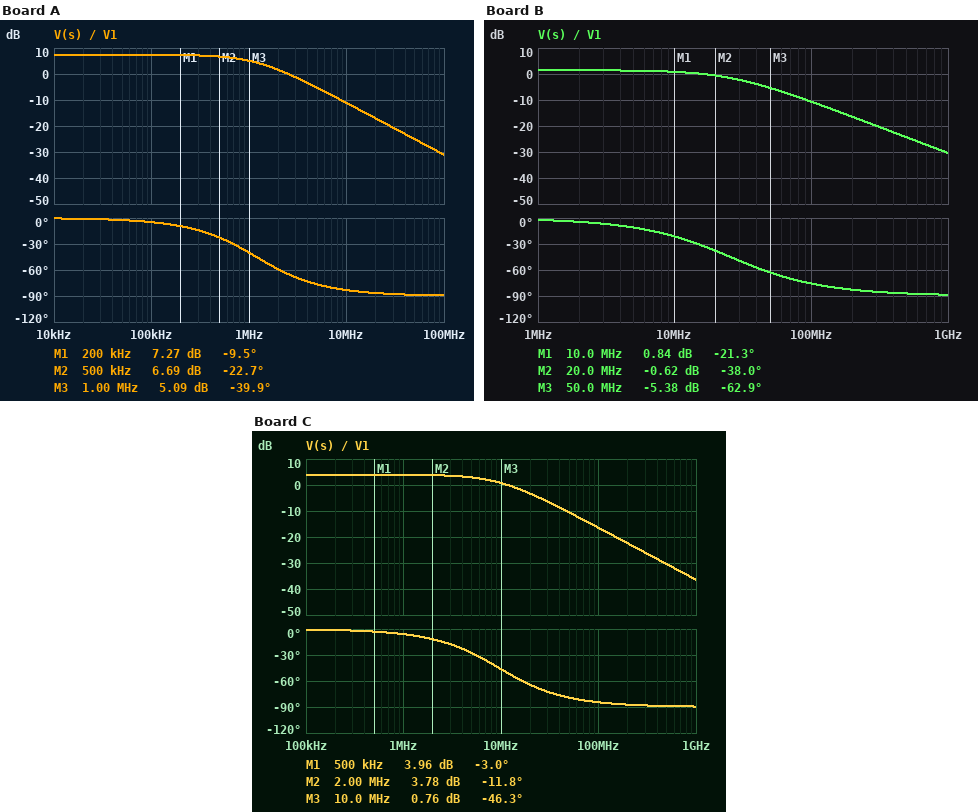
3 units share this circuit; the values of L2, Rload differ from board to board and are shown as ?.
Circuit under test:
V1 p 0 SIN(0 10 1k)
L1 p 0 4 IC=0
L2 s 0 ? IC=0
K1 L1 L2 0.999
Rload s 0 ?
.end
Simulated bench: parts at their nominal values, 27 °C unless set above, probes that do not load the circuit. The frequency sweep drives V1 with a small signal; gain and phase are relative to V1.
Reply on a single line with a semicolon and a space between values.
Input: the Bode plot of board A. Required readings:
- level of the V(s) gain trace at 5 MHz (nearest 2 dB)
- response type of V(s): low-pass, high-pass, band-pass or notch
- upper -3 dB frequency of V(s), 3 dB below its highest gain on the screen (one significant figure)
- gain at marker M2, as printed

-6 dB; low-pass; 1 MHz; 6.69 dB
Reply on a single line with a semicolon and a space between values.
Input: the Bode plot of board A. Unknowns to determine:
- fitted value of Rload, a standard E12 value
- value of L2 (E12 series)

330 kΩ; 22 H
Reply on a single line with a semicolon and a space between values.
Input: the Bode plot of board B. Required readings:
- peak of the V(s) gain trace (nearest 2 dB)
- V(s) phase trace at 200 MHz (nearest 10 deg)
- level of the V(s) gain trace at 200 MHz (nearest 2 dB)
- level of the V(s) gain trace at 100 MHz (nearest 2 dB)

2 dB; -80 deg; -16 dB; -10 dB
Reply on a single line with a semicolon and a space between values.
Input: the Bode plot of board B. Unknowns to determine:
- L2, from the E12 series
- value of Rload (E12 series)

5.6 H; 1.8 MΩ
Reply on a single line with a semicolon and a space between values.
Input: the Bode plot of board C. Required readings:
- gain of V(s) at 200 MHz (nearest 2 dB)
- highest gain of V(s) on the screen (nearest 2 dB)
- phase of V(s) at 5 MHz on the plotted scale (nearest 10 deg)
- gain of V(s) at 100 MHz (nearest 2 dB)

-22 dB; 4 dB; -30 deg; -16 dB
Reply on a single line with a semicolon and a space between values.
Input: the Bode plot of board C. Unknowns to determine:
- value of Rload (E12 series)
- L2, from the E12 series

1.2 MΩ; 10 H
